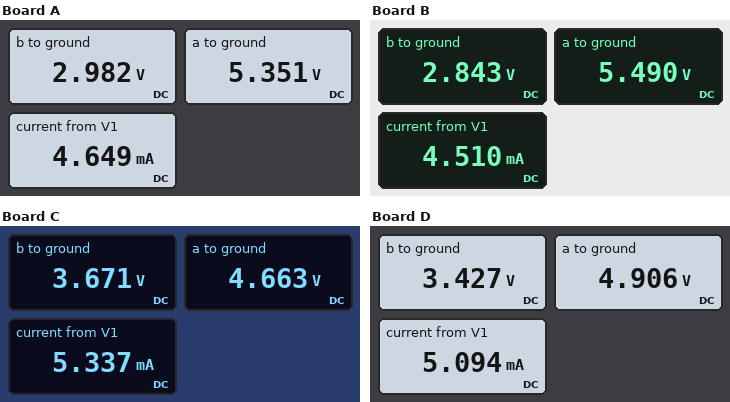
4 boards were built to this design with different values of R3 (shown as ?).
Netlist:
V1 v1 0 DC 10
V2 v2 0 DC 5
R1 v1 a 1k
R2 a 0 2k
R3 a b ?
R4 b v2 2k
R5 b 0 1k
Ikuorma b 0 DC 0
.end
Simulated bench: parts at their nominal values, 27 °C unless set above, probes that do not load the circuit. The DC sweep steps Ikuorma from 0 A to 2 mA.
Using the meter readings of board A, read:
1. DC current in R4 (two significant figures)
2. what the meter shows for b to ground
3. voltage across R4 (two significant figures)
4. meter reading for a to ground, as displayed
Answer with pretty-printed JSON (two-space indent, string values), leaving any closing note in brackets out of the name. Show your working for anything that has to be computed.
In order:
{
  "DC current in R4": "(5 V - 2.982 V) / 2 kΩ = 1.0 mA",
  "what the meter shows for b to ground": "2.982 V",
  "voltage across R4": "5 V - 2.982 V = 2.0 V",
  "meter reading for a to ground, as displayed": "5.351 V"
}
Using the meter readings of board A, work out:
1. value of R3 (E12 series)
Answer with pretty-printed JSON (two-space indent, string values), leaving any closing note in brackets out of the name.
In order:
{
  "value of R3": "1.2 kΩ"
}
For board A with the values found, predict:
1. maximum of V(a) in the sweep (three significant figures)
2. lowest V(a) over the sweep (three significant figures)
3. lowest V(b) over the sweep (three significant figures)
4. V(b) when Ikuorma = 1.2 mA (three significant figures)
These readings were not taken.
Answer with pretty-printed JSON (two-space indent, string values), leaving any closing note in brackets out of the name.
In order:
{
  "maximum of V(a) in the sweep": "5.35 V",
  "lowest V(a) over the sweep": "5.00 V",
  "lowest V(b) over the sweep": "2.00 V",
  "V(b) when Ikuorma = 1.2 mA": "2.39 V"
}
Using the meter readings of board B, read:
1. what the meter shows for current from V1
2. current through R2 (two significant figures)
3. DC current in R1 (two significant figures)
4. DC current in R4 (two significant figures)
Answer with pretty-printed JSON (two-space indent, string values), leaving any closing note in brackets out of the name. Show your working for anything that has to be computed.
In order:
{
  "what the meter shows for current from V1": "4.510 mA",
  "current through R2": "(5.49 V) / 2 kΩ = 2.7 mA",
  "DC current in R1": "(10 V - 5.49 V) / 1 kΩ = 4.5 mA",
  "DC current in R4": "(5 V - 2.843 V) / 2 kΩ = 1.1 mA"
}
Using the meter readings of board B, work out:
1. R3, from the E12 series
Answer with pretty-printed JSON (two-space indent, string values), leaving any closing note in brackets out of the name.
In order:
{
  "R3, from the E12 series": "1.5 kΩ"
}
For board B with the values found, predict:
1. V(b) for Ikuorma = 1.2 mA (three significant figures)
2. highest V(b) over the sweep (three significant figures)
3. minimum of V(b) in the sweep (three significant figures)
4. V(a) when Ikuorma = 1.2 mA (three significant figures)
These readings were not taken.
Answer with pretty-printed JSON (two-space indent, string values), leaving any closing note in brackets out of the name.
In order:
{
  "V(b) for Ikuorma = 1.2 mA": "2.23 V",
  "highest V(b) over the sweep": "2.84 V",
  "minimum of V(b) in the sweep": "1.82 V",
  "V(a) when Ikuorma = 1.2 mA": "5.30 V"
}
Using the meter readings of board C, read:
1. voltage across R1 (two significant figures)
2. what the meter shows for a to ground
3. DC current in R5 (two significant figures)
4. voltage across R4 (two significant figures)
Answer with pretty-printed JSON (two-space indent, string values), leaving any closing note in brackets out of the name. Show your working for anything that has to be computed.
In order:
{
  "voltage across R1": "10 V - 4.663 V = 5.3 V",
  "what the meter shows for a to ground": "4.663 V",
  "DC current in R5": "(3.671 V) / 1 kΩ = 3.7 mA",
  "voltage across R4": "5 V - 3.671 V = 1.3 V"
}
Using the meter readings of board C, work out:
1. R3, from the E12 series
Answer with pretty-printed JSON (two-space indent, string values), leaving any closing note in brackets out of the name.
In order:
{
  "R3, from the E12 series": "330 Ω"
}
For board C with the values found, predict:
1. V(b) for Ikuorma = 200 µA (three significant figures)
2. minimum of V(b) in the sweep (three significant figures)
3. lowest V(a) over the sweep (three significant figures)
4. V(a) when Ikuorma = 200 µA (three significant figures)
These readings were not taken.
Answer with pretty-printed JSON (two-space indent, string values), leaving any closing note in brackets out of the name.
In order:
{
  "V(b) for Ikuorma = 200 µA": "3.59 V",
  "minimum of V(b) in the sweep": "2.87 V",
  "lowest V(a) over the sweep": "4.13 V",
  "V(a) when Ikuorma = 200 µA": "4.61 V"
}
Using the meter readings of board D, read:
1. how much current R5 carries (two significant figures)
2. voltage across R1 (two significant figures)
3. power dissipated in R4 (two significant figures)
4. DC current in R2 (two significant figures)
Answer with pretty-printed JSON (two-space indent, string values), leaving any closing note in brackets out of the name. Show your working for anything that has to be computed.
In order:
{
  "how much current R5 carries": "(3.427 V) / 1 kΩ = 3.4 mA",
  "voltage across R1": "10 V - 4.906 V = 5.1 V",
  "power dissipated in R4": "(5 V - 3.427 V)^2 / 2 kΩ = 1.2 mW",
  "DC current in R2": "(4.906 V) / 2 kΩ = 2.5 mA"
}
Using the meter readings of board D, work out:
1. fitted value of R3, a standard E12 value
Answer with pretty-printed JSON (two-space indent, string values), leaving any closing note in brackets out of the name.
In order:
{
  "fitted value of R3, a standard E12 value": "560 Ω"
}
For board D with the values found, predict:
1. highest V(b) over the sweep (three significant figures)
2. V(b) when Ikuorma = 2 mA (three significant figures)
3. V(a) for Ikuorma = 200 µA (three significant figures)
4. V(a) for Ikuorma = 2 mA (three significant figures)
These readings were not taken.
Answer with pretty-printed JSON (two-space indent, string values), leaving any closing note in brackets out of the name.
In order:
{
  "highest V(b) over the sweep": "3.43 V",
  "V(b) when Ikuorma = 2 mA": "2.56 V",
  "V(a) for Ikuorma = 200 µA": "4.86 V",
  "V(a) for Ikuorma = 2 mA": "4.44 V"
}
